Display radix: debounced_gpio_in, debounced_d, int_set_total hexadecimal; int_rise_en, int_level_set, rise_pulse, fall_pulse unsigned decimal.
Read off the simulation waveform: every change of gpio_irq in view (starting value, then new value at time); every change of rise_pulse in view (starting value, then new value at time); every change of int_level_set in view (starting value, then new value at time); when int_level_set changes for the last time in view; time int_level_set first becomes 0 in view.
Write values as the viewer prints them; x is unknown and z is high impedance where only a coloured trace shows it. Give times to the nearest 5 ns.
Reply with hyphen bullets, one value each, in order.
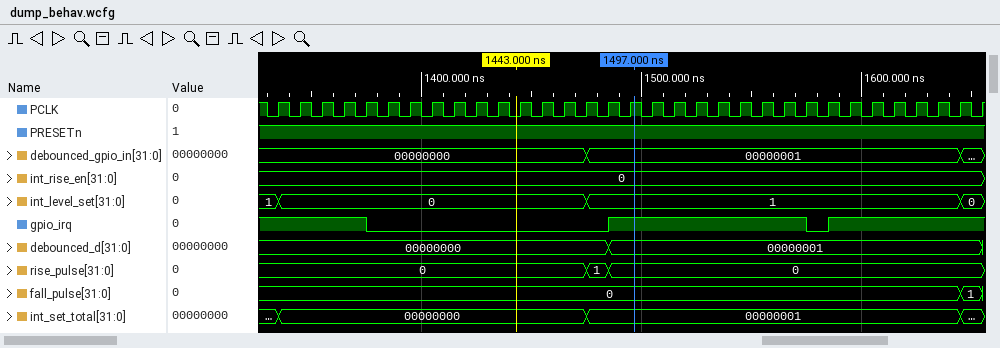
- 1, 0 at 1375 ns, 1 at 1485 ns, 0 at 1575 ns, 1 at 1585 ns
- 0, 1 at 1475 ns, 0 at 1485 ns
- 1, 0 at 1335 ns, 1 at 1475 ns, 0 at 1645 ns
- 1645 ns
- 1335 ns
